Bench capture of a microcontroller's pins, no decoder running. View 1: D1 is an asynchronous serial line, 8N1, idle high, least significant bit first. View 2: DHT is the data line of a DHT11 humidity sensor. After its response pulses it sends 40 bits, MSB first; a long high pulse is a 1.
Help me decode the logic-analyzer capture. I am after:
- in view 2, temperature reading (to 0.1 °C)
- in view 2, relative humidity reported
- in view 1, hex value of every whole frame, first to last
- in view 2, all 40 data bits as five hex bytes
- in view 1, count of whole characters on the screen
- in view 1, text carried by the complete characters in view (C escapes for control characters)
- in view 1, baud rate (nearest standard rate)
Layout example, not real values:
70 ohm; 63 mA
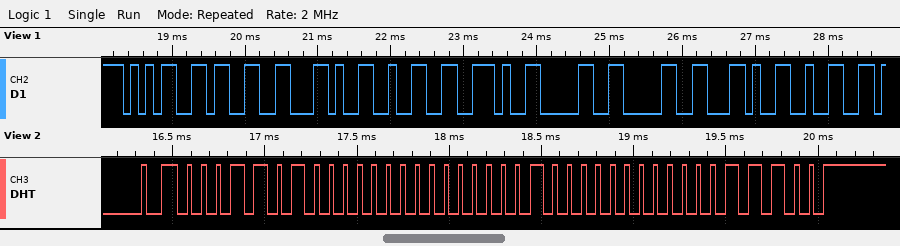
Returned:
2.0 °C; 26 %; 35 33 2C 32 2E 30 30 2C 32; 1A 00 02 00 1C; 9; "53,2.00,2"; 9600 baud
